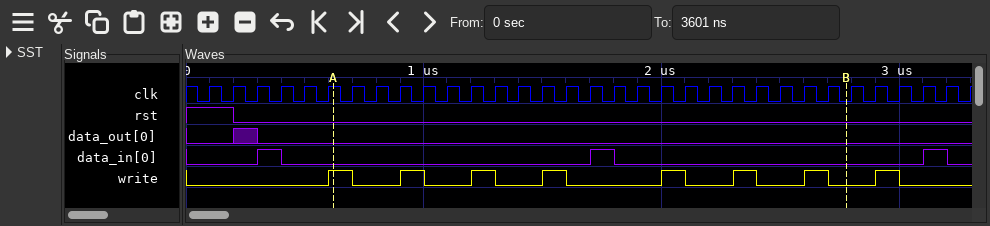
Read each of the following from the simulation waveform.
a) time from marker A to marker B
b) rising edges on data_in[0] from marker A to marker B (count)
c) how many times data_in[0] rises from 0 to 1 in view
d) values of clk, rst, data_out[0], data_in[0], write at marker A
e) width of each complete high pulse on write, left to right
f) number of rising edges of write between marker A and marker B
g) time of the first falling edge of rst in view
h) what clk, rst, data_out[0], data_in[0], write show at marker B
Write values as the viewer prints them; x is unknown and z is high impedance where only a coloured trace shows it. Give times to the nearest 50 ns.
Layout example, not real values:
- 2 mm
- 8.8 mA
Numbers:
- 2150 ns
- 1
- 3
- clk=1, rst=0, data_out[0]=0, data_in[0]=0, write=1
- 100 ns, 100 ns, 100 ns, 100 ns, 100 ns, 100 ns, 100 ns, 100 ns
- 6
- 200 ns
- clk=0, rst=0, data_out[0]=0, data_in[0]=0, write=0
